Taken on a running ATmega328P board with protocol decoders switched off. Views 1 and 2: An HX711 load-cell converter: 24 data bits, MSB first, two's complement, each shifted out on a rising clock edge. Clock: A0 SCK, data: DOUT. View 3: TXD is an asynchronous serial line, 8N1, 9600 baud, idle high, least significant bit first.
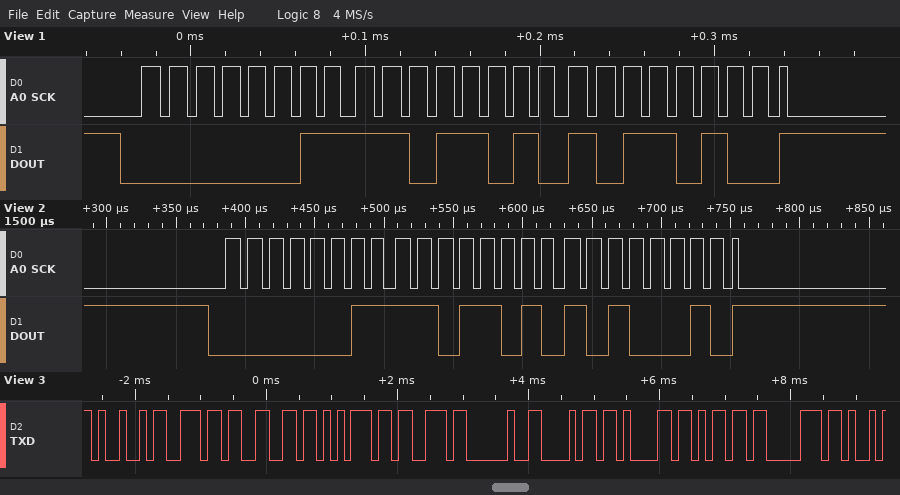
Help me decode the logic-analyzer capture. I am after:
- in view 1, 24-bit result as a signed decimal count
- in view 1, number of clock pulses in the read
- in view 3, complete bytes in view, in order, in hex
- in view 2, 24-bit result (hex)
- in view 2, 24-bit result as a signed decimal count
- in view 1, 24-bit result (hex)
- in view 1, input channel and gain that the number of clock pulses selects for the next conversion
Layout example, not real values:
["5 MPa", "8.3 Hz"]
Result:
["252596", "25", "49 6E 66 75 73 20 68 61 6D 70", "0x03DAA2", "252578", "0x03DAB4", "channel A, gain 128"]
